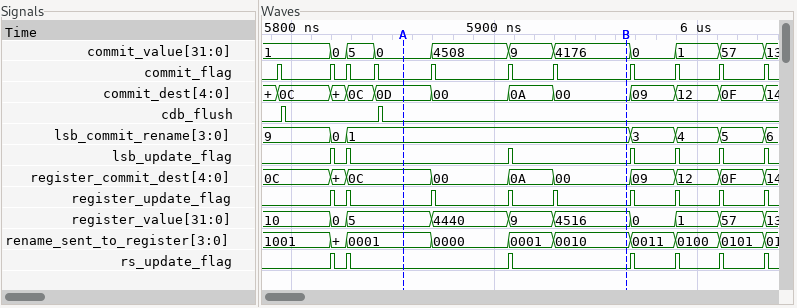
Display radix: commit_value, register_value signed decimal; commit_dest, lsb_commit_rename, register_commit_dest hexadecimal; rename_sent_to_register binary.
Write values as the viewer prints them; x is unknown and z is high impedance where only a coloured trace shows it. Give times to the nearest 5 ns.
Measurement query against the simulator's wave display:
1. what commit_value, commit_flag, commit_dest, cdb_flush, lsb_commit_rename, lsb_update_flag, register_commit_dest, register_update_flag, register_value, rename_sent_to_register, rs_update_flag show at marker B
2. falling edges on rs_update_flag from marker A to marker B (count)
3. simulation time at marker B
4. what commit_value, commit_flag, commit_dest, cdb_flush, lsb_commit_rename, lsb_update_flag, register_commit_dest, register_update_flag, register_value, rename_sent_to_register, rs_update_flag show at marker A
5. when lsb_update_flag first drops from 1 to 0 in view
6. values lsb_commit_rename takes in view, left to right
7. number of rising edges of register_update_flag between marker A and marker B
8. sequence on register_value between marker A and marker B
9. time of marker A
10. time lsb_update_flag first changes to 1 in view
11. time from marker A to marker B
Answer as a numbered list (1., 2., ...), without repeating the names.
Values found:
1. commit_value=4176, commit_flag=0, commit_dest=00, cdb_flush=0, lsb_commit_rename=1, lsb_update_flag=0, register_commit_dest=00, register_update_flag=0, register_value=4516, rename_sent_to_register=0010, rs_update_flag=0
2. 1
3. 5965 ns
4. commit_value=0, commit_flag=0, commit_dest=0D, cdb_flush=0, lsb_commit_rename=1, lsb_update_flag=0, register_commit_dest=0C, register_update_flag=0, register_value=5, rename_sent_to_register=0001, rs_update_flag=0
5. 5820 ns
6. 9, 0, 1, 3, 4, 5, 6
7. 3
8. 5, 4440, 9, 4516
9. 5855 ns
10. 5820 ns
11. 110 ns
